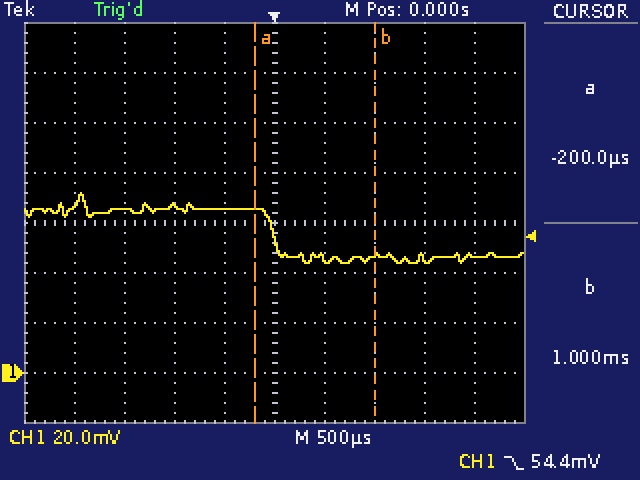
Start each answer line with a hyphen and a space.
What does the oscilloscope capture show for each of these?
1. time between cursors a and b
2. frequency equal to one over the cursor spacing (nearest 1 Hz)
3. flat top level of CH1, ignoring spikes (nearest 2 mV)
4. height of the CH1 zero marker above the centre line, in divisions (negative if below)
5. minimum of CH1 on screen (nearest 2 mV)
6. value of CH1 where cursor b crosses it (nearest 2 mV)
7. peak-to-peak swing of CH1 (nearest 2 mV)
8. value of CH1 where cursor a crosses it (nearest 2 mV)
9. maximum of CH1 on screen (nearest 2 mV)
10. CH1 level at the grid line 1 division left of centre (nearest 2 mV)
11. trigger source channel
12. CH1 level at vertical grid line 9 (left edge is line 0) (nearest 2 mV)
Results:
- 1.20 ms
- 833 Hz
- 66 mV
- -3.0 div
- 44 mV
- 46 mV
- 28 mV
- 66 mV
- 72 mV
- 66 mV
- CH1
- 46 mV
